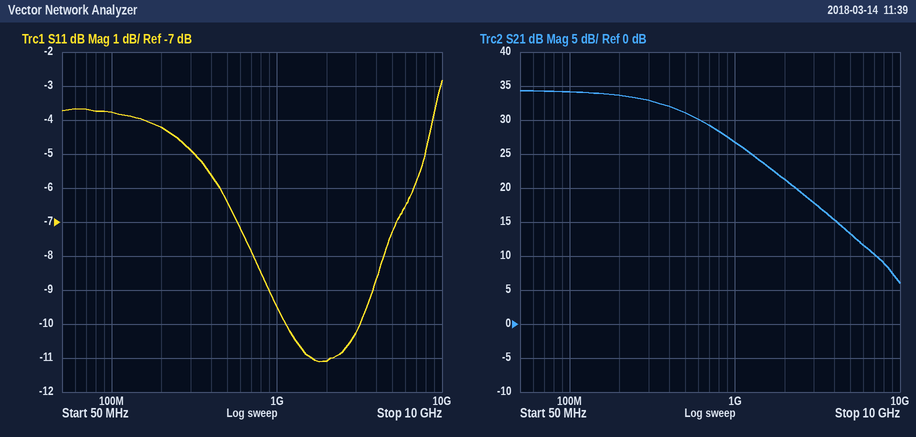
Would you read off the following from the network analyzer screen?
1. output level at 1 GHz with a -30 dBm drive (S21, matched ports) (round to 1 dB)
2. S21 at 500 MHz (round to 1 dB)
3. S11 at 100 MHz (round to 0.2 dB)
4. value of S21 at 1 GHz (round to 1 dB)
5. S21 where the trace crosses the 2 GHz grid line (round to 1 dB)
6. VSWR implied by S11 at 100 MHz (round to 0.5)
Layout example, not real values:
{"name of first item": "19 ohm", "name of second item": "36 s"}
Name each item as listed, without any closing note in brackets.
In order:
{"output level at 1 GHz with a -30 dBm drive (S21, matched ports)": "-3 dBm", "S21 at 500 MHz": "31 dB", "S11 at 100 MHz": "-3.8 dB", "value of S21 at 1 GHz": "27 dB", "S21 where the trace crosses the 2 GHz grid line": "21 dB", "VSWR implied by S11 at 100 MHz": "4.5"}
